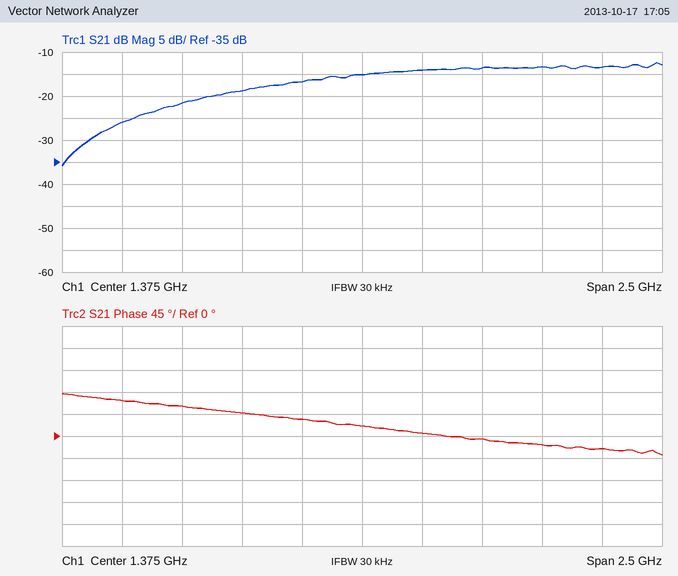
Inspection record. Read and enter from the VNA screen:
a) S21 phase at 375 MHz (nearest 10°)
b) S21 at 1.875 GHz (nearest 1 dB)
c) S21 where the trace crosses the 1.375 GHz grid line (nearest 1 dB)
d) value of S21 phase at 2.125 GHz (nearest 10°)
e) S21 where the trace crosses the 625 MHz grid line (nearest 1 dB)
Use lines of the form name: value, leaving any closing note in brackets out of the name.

S21 phase at 375 MHz: 70°
S21 at 1.875 GHz: -14 dB
S21 where the trace crosses the 1.375 GHz grid line: -15 dB
value of S21 phase at 2.125 GHz: -20°
S21 where the trace crosses the 625 MHz grid line: -22 dB
